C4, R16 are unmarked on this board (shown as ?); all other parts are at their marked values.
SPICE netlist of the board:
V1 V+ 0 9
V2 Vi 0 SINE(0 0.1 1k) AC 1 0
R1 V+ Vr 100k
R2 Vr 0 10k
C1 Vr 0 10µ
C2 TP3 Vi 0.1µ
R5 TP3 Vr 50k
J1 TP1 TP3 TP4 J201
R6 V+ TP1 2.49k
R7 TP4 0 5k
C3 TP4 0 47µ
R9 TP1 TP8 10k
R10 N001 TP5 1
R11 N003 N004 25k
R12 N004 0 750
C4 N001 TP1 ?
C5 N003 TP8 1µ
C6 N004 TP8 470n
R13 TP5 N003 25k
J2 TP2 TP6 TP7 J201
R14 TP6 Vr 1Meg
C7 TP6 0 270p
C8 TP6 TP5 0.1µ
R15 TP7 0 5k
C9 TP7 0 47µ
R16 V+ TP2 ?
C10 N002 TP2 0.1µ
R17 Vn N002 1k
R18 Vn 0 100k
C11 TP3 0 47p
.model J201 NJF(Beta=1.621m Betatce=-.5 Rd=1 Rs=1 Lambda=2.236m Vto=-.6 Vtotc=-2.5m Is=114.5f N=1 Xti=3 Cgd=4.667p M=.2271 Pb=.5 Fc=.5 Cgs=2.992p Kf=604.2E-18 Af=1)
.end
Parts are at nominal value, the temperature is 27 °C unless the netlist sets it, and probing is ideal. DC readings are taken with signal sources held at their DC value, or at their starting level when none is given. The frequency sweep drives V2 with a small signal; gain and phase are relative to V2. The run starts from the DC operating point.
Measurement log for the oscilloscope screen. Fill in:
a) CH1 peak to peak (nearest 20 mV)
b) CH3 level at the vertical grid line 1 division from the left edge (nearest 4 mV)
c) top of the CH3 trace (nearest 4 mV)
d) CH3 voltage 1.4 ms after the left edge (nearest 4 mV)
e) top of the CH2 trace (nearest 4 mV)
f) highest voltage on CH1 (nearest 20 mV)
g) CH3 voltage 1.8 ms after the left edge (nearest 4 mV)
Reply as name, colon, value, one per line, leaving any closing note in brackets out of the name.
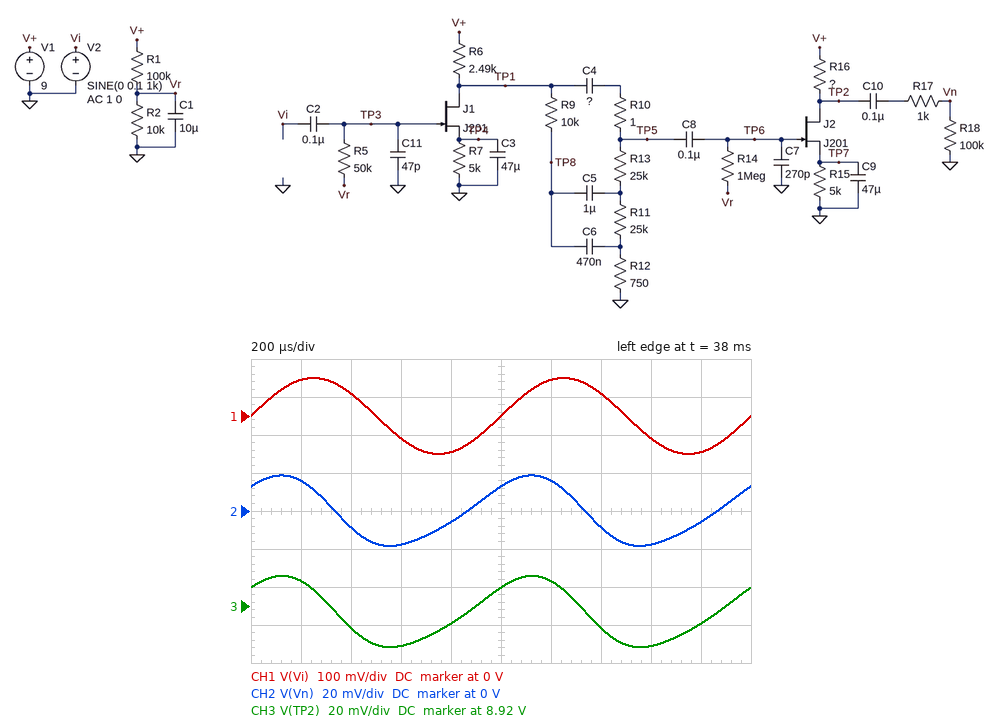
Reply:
CH1 peak to peak: 200 mV
CH3 level at the vertical grid line 1 division from the left edge: 8.932 V
top of the CH3 trace: 8.936 V
CH3 voltage 1.4 ms after the left edge: 8.908 V
top of the CH2 trace: 20 mV
highest voltage on CH1: 100 mV
CH3 voltage 1.8 ms after the left edge: 8.912 V
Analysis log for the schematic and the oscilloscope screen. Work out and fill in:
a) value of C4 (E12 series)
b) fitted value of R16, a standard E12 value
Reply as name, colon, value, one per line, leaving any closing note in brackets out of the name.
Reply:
value of C4: 1.2 nF
fitted value of R16, a standard E12 value: 390 Ω
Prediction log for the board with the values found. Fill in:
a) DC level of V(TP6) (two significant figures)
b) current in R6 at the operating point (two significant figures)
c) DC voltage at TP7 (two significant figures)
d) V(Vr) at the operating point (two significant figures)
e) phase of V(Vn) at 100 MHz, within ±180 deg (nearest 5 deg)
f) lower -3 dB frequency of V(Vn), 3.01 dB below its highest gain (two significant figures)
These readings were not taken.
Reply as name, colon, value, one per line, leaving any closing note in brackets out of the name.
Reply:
DC level of V(TP6): 820 mV
current in R6 at the operating point: 210 µA
DC voltage at TP7: 1.1 V
V(Vr) at the operating point: 820 mV
phase of V(Vn) at 100 MHz, within ±180 deg: -170 deg
lower -3 dB frequency of V(Vn), 3.01 dB below its highest gain: 4.1 kHz
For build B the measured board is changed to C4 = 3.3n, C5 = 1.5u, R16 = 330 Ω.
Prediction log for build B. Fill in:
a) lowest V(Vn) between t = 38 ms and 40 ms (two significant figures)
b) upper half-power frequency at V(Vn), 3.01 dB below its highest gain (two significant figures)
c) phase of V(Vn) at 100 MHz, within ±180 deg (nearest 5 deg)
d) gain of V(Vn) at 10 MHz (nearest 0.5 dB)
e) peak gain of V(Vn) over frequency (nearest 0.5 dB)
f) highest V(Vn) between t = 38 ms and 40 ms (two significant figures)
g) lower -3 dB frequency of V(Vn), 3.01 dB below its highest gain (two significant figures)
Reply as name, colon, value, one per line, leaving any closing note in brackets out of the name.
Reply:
lowest V(Vn) between t = 38 ms and 40 ms: -40 mV
upper half-power frequency at V(Vn), 3.01 dB below its highest gain: 330 kHz
phase of V(Vn) at 100 MHz, within ±180 deg: -165 deg
gain of V(Vn) at 10 MHz: -31.5 dB
peak gain of V(Vn) over frequency: -2.0 dB
highest V(Vn) between t = 38 ms and 40 ms: 37 mV
lower -3 dB frequency of V(Vn), 3.01 dB below its highest gain: 1.7 kHz
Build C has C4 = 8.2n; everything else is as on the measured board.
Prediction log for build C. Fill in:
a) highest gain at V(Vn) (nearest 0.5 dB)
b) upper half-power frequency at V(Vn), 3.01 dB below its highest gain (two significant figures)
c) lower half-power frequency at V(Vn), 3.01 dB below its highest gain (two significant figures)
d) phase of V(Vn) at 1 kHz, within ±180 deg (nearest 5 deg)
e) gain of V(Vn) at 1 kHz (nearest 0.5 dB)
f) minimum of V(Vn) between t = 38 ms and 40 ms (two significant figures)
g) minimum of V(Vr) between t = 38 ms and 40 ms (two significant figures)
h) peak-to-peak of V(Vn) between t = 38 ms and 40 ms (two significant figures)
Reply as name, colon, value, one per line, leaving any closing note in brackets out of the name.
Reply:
highest gain at V(Vn): 0 dB
upper half-power frequency at V(Vn), 3.01 dB below its highest gain: 320 kHz
lower half-power frequency at V(Vn), 3.01 dB below its highest gain: 760 Hz
phase of V(Vn) at 1 kHz, within ±180 deg: 35 deg
gain of V(Vn) at 1 kHz: -2.0 dB
minimum of V(Vn) between t = 38 ms and 40 ms: -79 mV
minimum of V(Vr) between t = 38 ms and 40 ms: 820 mV
peak-to-peak of V(Vn) between t = 38 ms and 40 ms: 150 mV
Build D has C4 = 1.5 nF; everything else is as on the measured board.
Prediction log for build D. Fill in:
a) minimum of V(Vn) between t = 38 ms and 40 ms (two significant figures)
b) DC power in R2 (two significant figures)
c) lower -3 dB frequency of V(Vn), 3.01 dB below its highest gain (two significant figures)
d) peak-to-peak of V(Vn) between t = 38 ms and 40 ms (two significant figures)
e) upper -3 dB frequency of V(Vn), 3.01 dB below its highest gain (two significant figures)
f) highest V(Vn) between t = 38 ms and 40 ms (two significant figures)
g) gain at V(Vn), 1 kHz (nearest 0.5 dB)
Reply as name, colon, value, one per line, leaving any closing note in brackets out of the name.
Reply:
minimum of V(Vn) between t = 38 ms and 40 ms: -23 mV
DC power in R2: 67 µW
lower -3 dB frequency of V(Vn), 3.01 dB below its highest gain: 3.4 kHz
peak-to-peak of V(Vn) between t = 38 ms and 40 ms: 46 mV
upper -3 dB frequency of V(Vn), 3.01 dB below its highest gain: 360 kHz
highest V(Vn) between t = 38 ms and 40 ms: 23 mV
gain at V(Vn), 1 kHz: -13.0 dB
